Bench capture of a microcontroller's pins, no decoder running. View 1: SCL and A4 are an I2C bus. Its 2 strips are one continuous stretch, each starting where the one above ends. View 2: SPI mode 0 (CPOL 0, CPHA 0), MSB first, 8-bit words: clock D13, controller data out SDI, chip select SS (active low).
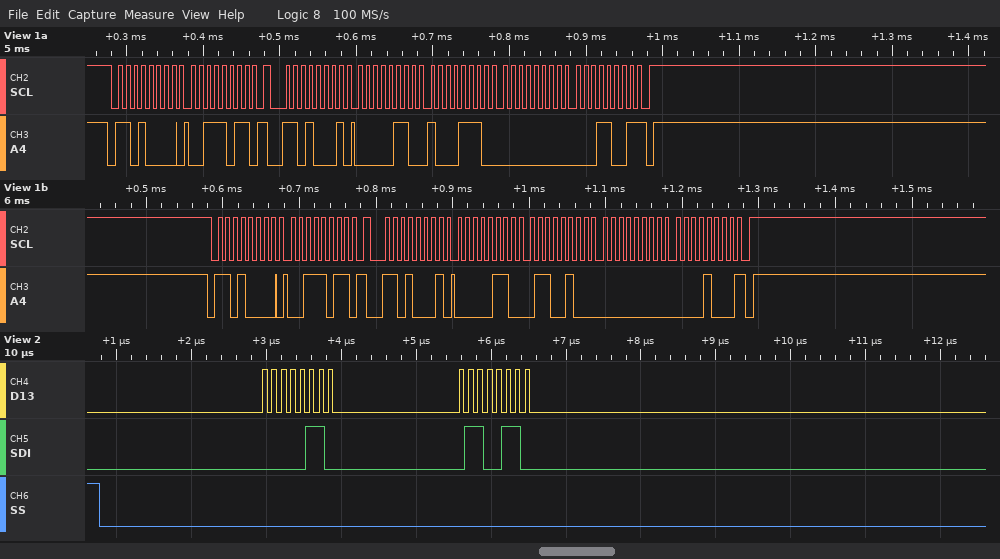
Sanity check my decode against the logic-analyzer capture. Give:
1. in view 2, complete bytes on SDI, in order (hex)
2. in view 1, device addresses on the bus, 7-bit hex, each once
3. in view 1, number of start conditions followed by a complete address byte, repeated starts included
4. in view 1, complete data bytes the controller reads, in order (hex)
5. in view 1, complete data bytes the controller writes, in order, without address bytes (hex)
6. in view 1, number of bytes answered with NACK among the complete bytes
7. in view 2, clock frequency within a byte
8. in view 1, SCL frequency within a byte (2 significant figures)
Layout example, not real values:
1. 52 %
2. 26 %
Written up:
1. 06 66
2. 0x68
3. 4
4. 06 8E 00 19 06 64 00 08
5. 3B 3B
6. 2
7. 8 MHz
8. 100 kHz
